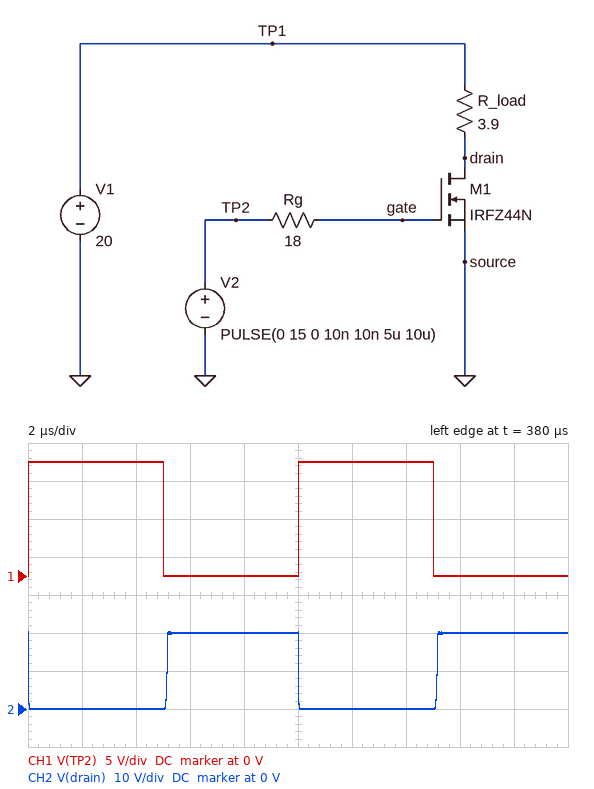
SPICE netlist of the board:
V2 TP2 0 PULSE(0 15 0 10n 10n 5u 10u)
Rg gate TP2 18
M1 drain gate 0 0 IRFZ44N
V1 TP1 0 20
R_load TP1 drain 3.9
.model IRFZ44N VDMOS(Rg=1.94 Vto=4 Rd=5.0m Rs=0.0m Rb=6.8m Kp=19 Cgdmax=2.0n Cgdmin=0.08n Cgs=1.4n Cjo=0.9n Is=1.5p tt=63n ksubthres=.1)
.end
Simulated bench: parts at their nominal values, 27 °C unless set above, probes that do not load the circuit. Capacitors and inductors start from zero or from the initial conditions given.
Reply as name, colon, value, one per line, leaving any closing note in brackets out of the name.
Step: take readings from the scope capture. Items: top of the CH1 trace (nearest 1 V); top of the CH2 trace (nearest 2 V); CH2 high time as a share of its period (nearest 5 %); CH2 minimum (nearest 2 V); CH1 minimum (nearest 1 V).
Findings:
top of the CH1 trace: 15 V
top of the CH2 trace: 20 V
CH2 high time as a share of its period: 50 %
CH2 minimum: 0 V
CH1 minimum: 0 V
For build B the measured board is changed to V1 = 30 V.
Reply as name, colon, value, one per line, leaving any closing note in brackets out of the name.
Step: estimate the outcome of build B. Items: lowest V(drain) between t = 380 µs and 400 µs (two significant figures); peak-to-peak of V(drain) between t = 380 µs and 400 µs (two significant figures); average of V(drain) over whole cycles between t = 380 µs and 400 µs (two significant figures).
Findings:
lowest V(drain) between t = 380 µs and 400 µs: 75 mV
peak-to-peak of V(drain) between t = 380 µs and 400 µs: 30 V
average of V(drain) over whole cycles between t = 380 µs and 400 µs: 15 V
